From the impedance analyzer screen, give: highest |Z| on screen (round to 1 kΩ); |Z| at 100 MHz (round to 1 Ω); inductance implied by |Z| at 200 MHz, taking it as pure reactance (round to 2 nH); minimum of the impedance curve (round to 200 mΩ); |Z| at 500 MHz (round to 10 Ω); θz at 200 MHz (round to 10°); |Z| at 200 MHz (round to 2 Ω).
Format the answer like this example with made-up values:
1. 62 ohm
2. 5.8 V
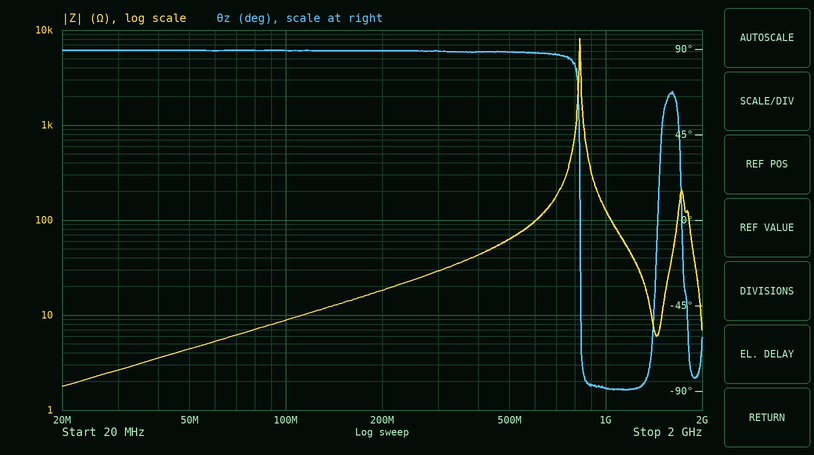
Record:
1. 8 kΩ
2. 9 Ω
3. 14 nH
4. 1.8 Ω
5. 60 Ω
6. 90°
7. 18 Ω
